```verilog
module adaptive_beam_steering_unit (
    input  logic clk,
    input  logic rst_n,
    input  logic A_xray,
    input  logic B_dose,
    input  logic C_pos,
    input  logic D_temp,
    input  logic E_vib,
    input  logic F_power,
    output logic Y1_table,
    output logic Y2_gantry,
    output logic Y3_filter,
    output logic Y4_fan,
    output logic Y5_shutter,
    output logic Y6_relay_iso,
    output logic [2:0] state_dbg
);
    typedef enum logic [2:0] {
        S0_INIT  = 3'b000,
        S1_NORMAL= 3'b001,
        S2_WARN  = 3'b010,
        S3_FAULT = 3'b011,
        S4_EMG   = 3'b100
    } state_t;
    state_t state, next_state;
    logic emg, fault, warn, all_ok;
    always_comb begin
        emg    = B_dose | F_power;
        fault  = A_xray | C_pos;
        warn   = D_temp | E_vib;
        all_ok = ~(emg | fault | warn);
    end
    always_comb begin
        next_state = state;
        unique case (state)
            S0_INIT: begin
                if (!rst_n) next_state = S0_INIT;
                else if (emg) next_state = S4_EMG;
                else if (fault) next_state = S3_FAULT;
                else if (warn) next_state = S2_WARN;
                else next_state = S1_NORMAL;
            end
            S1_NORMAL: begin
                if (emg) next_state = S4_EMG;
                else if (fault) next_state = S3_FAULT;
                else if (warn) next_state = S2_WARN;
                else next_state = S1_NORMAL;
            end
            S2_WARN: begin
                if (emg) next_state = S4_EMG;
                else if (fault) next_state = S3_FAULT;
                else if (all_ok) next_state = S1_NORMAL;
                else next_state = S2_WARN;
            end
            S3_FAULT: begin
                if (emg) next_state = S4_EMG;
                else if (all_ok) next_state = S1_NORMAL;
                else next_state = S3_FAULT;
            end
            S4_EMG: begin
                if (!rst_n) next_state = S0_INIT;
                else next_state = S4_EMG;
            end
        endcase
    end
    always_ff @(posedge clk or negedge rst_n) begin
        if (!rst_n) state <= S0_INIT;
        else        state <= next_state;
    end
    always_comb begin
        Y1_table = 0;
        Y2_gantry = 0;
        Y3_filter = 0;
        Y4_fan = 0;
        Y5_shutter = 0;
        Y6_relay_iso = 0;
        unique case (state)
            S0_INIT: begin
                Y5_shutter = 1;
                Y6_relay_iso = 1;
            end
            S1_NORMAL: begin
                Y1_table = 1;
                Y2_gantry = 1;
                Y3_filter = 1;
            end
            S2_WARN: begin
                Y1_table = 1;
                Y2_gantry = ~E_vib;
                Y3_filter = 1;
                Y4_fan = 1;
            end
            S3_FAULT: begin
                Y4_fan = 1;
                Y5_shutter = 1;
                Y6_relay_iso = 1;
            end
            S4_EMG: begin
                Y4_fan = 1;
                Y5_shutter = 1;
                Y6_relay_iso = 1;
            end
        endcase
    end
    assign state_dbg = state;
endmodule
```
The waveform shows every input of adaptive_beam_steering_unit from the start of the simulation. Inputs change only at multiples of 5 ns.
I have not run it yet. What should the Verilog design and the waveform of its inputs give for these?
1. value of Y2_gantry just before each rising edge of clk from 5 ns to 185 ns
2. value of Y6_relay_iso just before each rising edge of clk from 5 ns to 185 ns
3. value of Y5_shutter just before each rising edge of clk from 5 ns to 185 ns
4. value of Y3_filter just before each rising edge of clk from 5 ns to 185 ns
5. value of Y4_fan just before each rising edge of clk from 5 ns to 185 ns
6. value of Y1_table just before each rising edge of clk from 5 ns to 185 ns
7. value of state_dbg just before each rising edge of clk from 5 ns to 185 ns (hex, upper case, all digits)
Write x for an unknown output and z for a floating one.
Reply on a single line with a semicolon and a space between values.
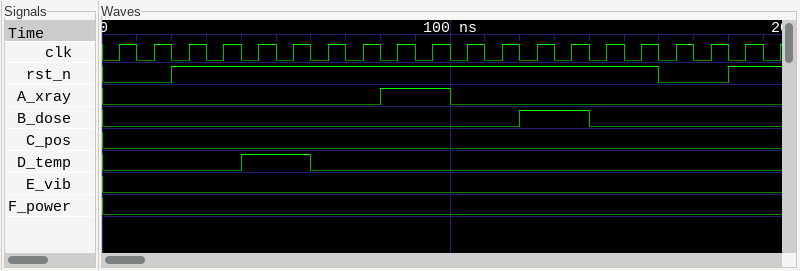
0 0 0 1 1 1 1 1 1 0 0 1 1 0 0 0 0 0 0; 1 1 1 0 0 0 0 0 0 1 1 0 0 1 1 1 1 1 1; 1 1 1 0 0 0 0 0 0 1 1 0 0 1 1 1 1 1 1; 0 0 0 1 1 1 1 1 1 0 0 1 1 0 0 0 0 0 0; 0 0 0 0 0 1 1 0 0 1 1 0 0 1 1 1 0 0 0; 0 0 0 1 1 1 1 1 1 0 0 1 1 0 0 0 0 0 0; 0, 0, 0, 1, 1, 2, 2, 1, 1, 3, 3, 1, 1, 4, 4, 4, 0, 0, 0
